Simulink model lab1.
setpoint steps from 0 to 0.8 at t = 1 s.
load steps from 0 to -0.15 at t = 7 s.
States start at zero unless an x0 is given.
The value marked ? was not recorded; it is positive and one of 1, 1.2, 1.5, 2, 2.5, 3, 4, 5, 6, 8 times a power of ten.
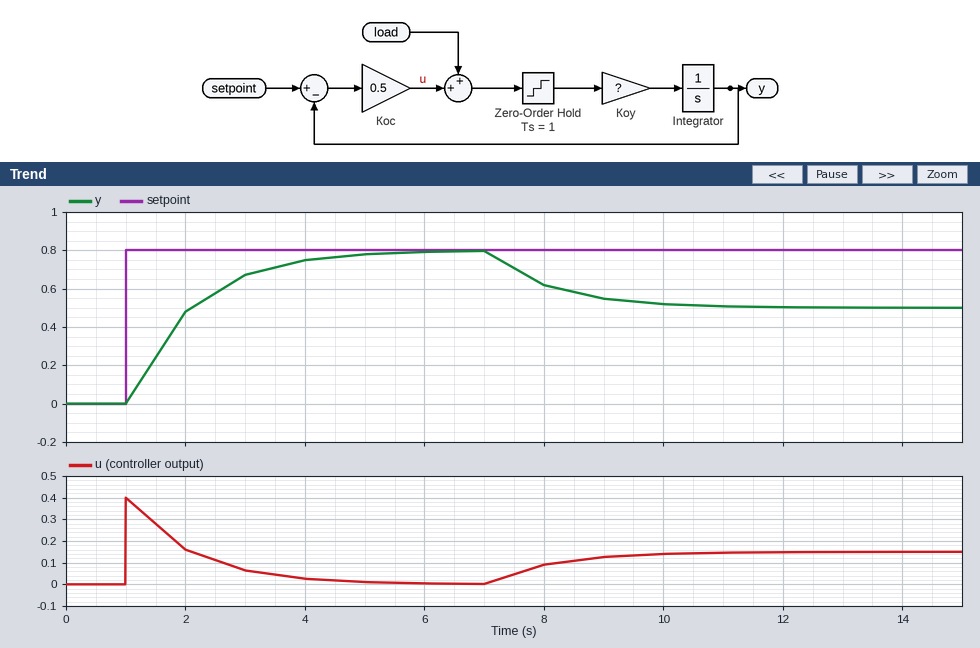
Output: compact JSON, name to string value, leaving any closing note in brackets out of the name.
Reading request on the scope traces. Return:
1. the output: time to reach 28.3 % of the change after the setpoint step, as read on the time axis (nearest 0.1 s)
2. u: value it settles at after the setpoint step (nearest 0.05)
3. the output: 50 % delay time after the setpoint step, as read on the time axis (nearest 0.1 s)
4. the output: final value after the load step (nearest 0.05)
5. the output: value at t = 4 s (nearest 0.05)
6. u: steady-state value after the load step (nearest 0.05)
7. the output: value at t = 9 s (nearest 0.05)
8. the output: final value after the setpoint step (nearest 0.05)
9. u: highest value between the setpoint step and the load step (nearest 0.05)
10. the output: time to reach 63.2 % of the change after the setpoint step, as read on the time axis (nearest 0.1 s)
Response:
{"the output: time to reach 28.3 % of the change after the setpoint step, as read on the time axis": "1.5 s", "u: value it settles at after the setpoint step": "0.00", "the output: 50 % delay time after the setpoint step, as read on the time axis": "1.8 s", "the output: final value after the load step": "0.50", "the output: value at t = 4 s": "0.75", "u: steady-state value after the load step": "0.15", "the output: value at t = 9 s": "0.55", "the output: final value after the setpoint step": "0.80", "u: highest value between the setpoint step and the load step": "0.40", "the output: time to reach 63.2 % of the change after the setpoint step, as read on the time axis": "2.1 s"}
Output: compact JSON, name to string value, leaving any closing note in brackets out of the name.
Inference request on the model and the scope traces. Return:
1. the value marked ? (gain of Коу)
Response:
{"the value marked ?": "1.2"}
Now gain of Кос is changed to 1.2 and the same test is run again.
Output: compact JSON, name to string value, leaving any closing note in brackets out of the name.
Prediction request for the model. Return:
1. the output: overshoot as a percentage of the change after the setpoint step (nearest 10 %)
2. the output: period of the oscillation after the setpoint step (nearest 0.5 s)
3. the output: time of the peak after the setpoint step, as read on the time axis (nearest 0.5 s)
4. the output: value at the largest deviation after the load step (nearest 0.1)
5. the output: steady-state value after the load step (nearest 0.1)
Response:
{"the output: overshoot as a percentage of the change after the setpoint step": "40 %", "the output: period of the oscillation after the setpoint step": "2.0 s", "the output: time of the peak after the setpoint step, as read on the time axis": "2.0 s", "the output: value at the largest deviation after the load step": "0.6", "the output: steady-state value after the load step": "0.7"}
